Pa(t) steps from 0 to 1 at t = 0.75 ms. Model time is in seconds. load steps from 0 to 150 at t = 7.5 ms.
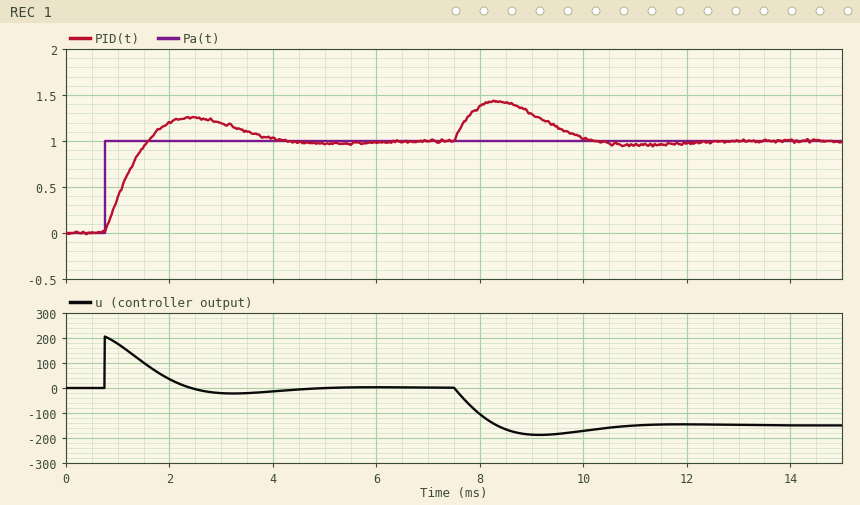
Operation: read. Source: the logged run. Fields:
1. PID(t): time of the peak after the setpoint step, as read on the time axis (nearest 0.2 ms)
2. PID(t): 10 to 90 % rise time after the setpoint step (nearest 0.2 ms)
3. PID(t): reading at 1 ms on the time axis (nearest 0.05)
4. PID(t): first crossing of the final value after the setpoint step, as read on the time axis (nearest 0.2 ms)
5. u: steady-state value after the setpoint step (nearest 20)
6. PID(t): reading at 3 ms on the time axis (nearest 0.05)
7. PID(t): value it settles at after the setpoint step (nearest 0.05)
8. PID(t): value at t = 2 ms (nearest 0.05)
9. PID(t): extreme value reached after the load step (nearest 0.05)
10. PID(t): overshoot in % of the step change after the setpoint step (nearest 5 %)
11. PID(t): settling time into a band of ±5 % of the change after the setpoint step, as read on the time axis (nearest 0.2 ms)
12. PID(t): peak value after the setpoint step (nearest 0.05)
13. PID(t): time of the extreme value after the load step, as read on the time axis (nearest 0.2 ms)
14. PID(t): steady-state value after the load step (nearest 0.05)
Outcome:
2.4 ms
0.6 ms
0.40
1.6 ms
0
1.20
1.00
1.20
1.45
25 %
3.8 ms
1.25
8.4 ms
1.00
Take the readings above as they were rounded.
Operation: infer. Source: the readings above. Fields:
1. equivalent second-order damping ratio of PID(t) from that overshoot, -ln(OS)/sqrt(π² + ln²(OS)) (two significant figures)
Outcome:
0.40
